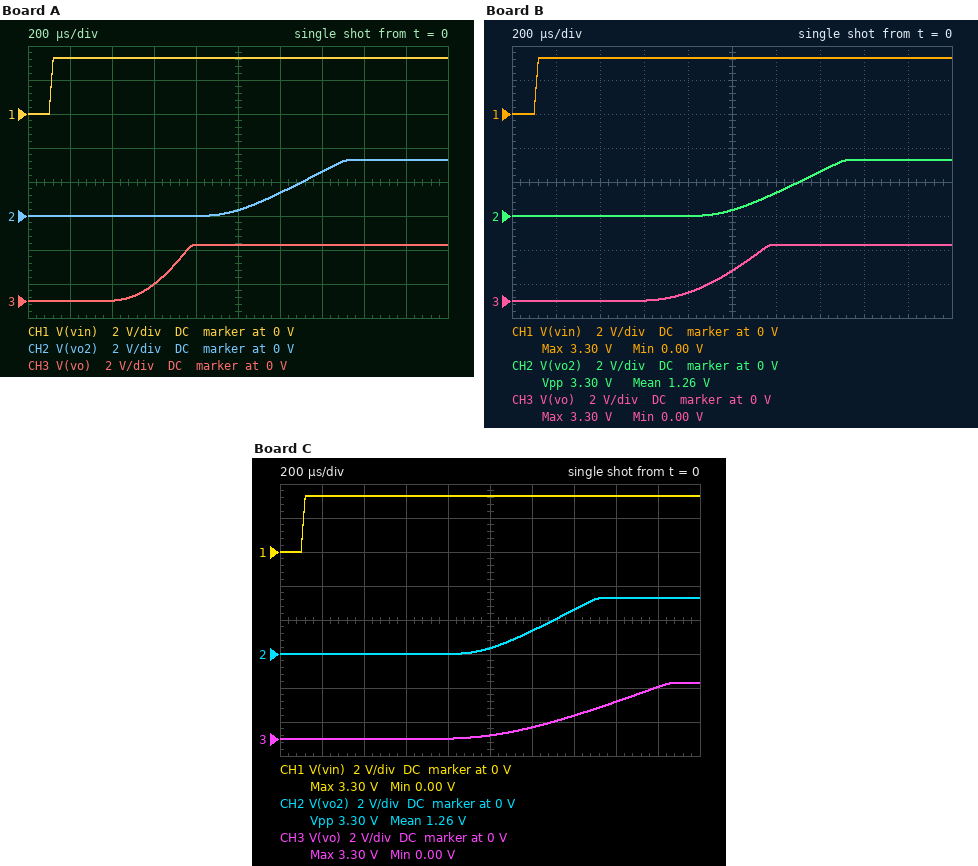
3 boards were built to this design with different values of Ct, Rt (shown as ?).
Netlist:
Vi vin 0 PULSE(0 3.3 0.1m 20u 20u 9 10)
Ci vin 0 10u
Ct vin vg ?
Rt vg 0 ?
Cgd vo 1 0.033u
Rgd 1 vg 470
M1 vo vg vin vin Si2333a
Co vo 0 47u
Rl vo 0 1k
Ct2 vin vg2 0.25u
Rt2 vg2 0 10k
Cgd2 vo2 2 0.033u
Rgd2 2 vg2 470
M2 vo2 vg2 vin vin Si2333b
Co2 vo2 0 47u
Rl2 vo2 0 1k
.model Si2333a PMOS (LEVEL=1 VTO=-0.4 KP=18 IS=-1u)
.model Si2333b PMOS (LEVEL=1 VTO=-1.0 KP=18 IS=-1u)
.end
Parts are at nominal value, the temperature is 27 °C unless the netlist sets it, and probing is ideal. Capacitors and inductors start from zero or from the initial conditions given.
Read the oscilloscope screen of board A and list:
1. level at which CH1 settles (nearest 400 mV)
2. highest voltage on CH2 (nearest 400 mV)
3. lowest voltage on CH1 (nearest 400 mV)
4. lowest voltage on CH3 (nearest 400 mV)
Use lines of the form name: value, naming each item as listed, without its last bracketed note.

level at which CH1 settles: 3.2 V
highest voltage on CH2: 3.2 V
lowest voltage on CH1: 0 V
lowest voltage on CH3: 0 V
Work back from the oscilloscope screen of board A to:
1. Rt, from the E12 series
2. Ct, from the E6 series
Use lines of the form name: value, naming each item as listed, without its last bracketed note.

Rt, from the E12 series: 3.9 kΩ
Ct, from the E6 series: 680 nF
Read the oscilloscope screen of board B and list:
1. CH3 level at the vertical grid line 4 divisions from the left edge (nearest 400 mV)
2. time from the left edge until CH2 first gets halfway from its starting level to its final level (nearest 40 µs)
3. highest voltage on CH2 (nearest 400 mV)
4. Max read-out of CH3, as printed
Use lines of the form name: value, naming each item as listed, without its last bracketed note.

CH3 level at the vertical grid line 4 divisions from the left edge: 400 mV
time from the left edge until CH2 first gets halfway from its starting level to its final level: 1.24 ms
highest voltage on CH2: 3.2 V
Max read-out of CH3, as printed: 3.30 V
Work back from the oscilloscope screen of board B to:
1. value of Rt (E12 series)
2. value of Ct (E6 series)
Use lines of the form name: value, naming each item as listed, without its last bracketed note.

value of Rt: 6.8 kΩ
value of Ct: 680 nF
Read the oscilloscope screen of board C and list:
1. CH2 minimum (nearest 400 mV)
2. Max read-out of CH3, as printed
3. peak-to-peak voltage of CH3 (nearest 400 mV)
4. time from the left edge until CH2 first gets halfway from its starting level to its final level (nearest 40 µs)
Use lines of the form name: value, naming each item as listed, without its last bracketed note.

CH2 minimum: 0 V
Max read-out of CH3, as printed: 3.30 V
peak-to-peak voltage of CH3: 3.2 V
time from the left edge until CH2 first gets halfway from its starting level to its final level: 1.24 ms
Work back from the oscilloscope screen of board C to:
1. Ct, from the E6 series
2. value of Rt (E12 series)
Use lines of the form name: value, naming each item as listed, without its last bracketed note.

Ct, from the E6 series: 470 nF
value of Rt: 18 kΩ
